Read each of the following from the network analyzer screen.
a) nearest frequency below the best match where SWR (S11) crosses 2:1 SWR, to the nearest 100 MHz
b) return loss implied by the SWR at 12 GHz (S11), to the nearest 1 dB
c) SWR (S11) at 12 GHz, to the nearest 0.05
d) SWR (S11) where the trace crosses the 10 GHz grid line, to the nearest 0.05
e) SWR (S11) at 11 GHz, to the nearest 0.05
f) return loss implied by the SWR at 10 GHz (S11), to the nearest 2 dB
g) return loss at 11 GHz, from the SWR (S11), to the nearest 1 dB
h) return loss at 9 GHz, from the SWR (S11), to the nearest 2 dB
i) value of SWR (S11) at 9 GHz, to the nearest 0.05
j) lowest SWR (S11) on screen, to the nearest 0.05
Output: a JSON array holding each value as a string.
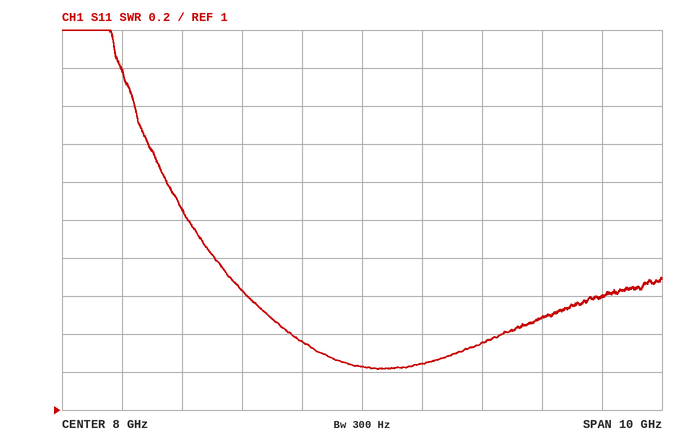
["5.1 GHz", "13 dB", "1.60", "1.35", "1.50", "16 dB", "14 dB", "20 dB", "1.25", "1.20"]
